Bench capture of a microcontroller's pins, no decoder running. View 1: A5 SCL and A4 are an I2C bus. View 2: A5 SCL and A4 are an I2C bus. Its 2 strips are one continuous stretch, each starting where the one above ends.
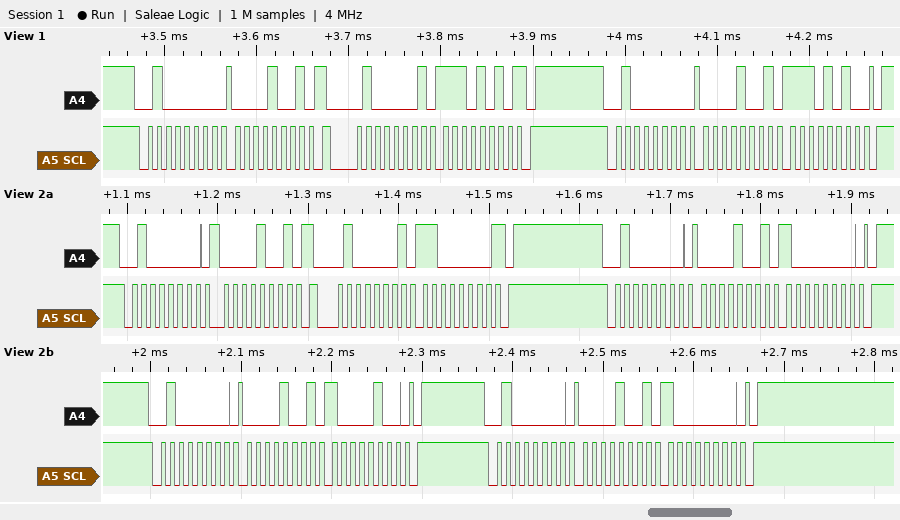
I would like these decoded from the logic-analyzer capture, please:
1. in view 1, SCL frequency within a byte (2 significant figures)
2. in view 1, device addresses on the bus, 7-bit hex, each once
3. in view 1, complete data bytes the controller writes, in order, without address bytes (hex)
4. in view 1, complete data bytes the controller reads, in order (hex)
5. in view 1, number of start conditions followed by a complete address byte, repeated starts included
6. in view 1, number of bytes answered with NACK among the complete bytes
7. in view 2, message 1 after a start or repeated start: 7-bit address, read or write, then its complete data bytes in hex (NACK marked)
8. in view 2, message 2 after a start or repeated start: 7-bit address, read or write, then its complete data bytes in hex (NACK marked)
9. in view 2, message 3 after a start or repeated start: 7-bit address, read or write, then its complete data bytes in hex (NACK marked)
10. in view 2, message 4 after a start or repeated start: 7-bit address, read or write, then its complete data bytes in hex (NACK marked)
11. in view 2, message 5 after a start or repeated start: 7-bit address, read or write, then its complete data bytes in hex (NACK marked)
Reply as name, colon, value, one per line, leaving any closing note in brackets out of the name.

in view 1, SCL frequency within a byte: 100 kHz
in view 1, device addresses on the bus, 7-bit hex, each once: 0x20
in view 1, complete data bytes the controller writes, in order, without address bytes: 09 09 EA
in view 1, complete data bytes the controller reads, in order: EA
in view 1, number of start conditions followed by a complete address byte, repeated starts included: 3
in view 1, number of bytes answered with NACK among the complete bytes: 1
in view 2, message 1 after a start or repeated start: 7-bit address, read or write, then its complete data bytes in hex: 0x20 write: 09
in view 2, message 2 after a start or repeated start: 7-bit address, read or write, then its complete data bytes in hex: 0x20 read: C0 NACK
in view 2, message 3 after a start or repeated start: 7-bit address, read or write, then its complete data bytes in hex: 0x20 write: 09 80
in view 2, message 4 after a start or repeated start: 7-bit address, read or write, then its complete data bytes in hex: 0x20 write: 09 84
in view 2, message 5 after a start or repeated start: 7-bit address, read or write, then its complete data bytes in hex: 0x20 write: 09 80
